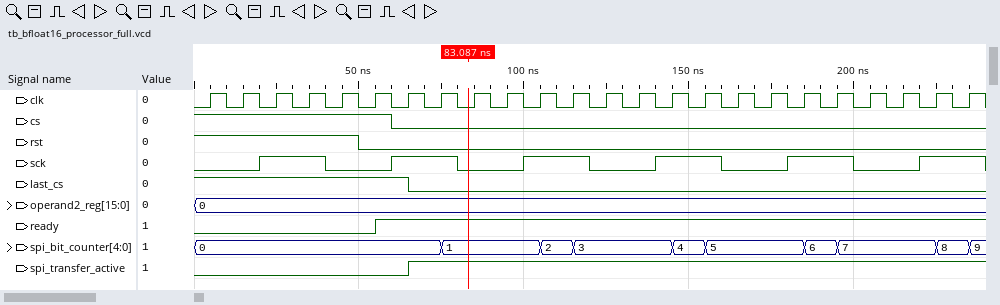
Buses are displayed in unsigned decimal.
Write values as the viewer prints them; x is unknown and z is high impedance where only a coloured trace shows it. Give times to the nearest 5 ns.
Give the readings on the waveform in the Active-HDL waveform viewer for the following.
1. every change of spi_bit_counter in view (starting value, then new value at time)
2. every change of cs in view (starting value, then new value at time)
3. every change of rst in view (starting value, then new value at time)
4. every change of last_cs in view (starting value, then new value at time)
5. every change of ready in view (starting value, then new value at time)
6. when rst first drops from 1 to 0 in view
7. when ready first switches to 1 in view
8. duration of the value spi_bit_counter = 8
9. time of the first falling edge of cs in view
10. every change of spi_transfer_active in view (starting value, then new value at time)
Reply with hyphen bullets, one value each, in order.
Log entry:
- 0, 1 at 75 ns, 2 at 105 ns, 3 at 115 ns, 4 at 145 ns, 5 at 155 ns, 6 at 185 ns, 7 at 195 ns, 8 at 225 ns, 9 at 235 ns
- 1, 0 at 60 ns
- 1, 0 at 50 ns
- 1, 0 at 65 ns
- 0, 1 at 55 ns
- 50 ns
- 55 ns
- 10 ns
- 60 ns
- 0, 1 at 65 ns
